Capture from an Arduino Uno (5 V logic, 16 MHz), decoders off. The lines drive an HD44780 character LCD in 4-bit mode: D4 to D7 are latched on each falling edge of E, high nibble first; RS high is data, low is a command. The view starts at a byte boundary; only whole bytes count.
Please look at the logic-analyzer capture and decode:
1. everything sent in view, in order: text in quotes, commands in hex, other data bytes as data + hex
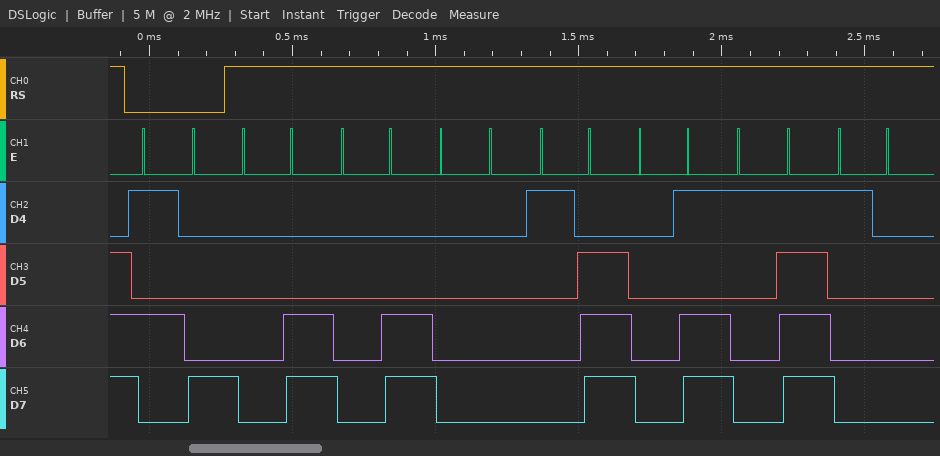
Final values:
0x58 data 0C 0C 00 1E 0D 1F 10
